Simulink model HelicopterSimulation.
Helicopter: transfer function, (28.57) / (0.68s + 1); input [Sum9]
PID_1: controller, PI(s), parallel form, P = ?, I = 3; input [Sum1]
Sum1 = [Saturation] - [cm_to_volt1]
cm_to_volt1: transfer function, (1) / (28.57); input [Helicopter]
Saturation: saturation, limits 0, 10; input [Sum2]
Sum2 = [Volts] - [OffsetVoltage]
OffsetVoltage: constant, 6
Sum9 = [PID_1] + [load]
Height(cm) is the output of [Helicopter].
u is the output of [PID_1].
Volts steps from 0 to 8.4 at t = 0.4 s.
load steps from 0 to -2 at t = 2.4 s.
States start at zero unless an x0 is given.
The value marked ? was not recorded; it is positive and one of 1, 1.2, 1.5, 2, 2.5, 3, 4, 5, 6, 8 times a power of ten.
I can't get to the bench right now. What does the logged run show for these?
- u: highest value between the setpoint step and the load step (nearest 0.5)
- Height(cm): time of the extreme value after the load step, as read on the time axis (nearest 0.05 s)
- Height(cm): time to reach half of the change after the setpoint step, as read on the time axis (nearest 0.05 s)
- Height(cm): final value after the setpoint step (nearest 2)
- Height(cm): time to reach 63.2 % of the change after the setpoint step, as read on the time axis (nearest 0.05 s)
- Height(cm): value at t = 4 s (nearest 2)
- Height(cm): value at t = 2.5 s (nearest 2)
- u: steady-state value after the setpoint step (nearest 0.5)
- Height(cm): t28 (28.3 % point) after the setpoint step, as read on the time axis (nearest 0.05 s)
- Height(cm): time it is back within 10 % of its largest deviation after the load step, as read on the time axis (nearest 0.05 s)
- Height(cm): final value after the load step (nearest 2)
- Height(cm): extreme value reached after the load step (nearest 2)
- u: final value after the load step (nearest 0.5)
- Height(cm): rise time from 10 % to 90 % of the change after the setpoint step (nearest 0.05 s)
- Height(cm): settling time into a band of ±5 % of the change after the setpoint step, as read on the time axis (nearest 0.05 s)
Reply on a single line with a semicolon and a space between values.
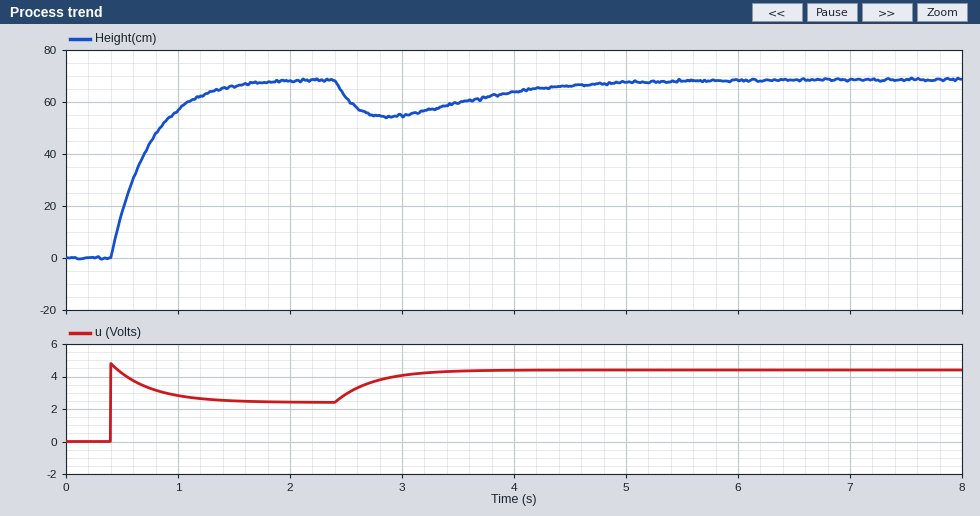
5.0; 2.85 s; 0.65 s; 68; 0.75 s; 64; 62; 2.5; 0.50 s; 4.85 s; 68; 54; 4.5; 0.75 s; 1.40 s
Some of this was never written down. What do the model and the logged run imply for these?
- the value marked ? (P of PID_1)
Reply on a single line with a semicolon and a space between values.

2
